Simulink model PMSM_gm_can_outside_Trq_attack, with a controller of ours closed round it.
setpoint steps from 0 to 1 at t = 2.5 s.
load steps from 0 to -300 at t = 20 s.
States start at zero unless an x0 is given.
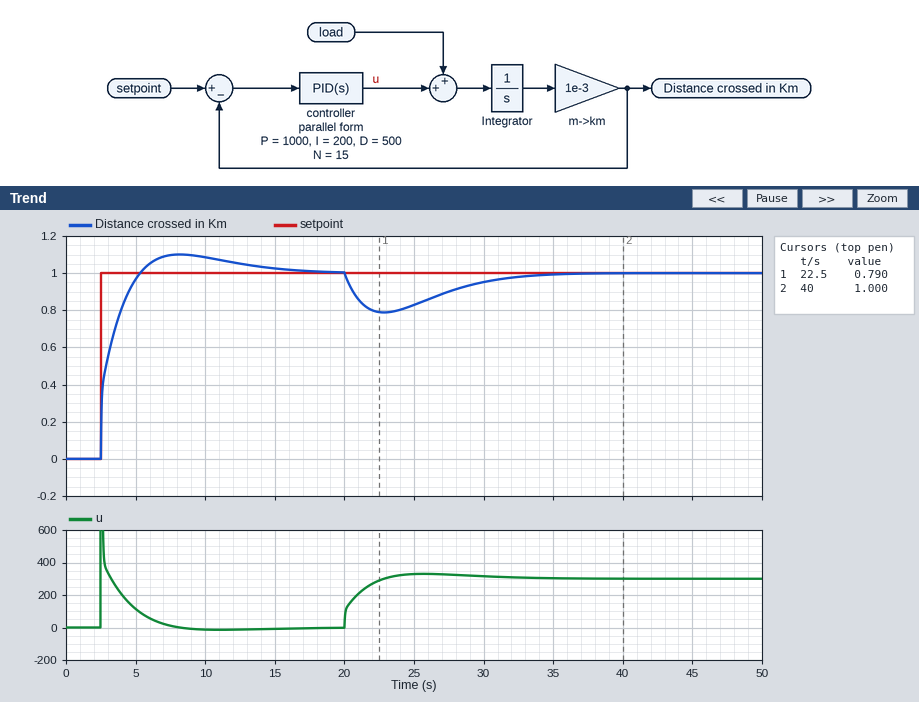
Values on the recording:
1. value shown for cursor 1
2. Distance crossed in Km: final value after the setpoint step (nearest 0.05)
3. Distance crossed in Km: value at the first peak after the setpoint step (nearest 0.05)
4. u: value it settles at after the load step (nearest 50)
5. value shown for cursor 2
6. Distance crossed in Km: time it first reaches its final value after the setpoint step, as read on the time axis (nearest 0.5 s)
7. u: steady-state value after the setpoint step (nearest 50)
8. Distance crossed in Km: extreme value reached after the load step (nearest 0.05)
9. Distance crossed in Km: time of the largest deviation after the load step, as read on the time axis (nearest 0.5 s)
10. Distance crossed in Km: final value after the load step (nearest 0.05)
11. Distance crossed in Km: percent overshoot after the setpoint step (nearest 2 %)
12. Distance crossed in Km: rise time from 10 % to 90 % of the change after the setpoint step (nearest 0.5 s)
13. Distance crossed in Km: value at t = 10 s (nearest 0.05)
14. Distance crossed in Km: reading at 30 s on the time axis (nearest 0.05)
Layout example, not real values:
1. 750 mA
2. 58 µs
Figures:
1. 0.790
2. 1.00
3. 1.10
4. 300
5. 1.000
6. 5.5 s
7. 0
8. 0.80
9. 23.0 s
10. 1.00
11. 10 %
12. 2.0 s
13. 1.10
14. 0.95
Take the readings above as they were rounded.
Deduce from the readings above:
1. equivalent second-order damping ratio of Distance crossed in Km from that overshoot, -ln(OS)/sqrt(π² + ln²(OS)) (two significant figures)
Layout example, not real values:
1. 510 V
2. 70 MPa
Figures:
1. 0.59
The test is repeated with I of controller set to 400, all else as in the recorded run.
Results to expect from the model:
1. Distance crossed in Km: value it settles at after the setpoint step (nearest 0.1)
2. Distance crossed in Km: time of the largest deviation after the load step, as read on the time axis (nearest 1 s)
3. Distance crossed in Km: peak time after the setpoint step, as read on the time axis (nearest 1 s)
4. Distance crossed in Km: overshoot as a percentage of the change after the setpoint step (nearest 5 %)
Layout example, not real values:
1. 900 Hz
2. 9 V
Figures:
1. 1.0
2. 22 s
3. 7 s
4. 15 %
